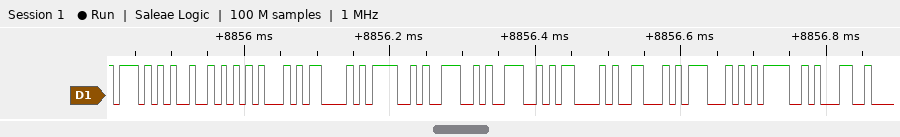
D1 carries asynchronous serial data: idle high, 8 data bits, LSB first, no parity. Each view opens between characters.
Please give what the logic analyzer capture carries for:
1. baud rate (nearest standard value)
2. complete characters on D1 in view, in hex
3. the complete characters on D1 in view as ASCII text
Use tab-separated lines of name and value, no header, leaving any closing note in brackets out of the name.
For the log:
baud rate	115200 baud
complete characters on D1 in view, in hex	57, 52, 45, 43, 4F, 4E, 4E, 43, 46, 47, 3D, 31
the complete characters on D1 in view as ASCII text	"WRECONNCFG=1"
